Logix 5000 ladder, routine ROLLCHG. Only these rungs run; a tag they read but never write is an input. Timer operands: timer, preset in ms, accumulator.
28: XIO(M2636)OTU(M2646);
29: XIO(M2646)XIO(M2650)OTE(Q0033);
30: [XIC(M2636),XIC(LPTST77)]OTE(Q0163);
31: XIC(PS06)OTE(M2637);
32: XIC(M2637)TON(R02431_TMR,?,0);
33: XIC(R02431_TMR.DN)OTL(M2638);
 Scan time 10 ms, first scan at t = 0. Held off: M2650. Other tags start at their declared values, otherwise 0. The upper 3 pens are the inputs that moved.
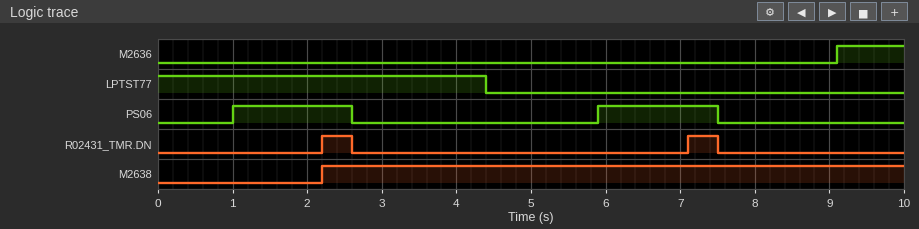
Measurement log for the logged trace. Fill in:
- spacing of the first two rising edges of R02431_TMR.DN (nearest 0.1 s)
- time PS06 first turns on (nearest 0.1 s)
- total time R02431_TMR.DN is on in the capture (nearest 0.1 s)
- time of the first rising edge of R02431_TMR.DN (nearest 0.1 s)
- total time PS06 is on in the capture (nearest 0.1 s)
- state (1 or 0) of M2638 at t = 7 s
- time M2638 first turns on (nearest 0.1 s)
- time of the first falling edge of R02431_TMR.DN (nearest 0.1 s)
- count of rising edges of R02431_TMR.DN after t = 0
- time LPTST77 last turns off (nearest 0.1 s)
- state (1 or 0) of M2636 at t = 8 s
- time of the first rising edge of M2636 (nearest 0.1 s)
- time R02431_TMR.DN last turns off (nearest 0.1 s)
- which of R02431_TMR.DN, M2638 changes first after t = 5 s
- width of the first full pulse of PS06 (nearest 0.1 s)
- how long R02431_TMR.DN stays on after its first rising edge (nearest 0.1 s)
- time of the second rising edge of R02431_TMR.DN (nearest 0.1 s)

4.9 s
1.0 s
0.8 s
2.2 s
3.2 s
1
2.2 s
2.6 s
2
4.4 s
0
9.1 s
7.5 s
R02431_TMR.DN
1.6 s
0.4 s
7.1 s
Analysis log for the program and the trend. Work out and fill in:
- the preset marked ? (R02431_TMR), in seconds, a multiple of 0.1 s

1.2 s
